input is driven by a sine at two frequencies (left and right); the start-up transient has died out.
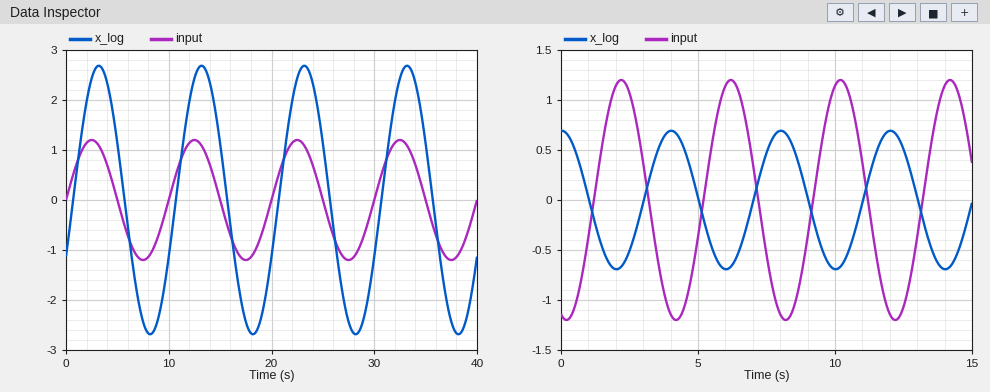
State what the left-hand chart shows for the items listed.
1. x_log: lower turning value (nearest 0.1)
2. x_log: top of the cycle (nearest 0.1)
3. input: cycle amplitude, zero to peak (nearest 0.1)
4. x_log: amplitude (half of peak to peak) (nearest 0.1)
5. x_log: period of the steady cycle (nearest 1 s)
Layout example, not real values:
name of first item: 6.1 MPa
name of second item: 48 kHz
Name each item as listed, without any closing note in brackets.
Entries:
x_log: lower turning value: -2.7
x_log: top of the cycle: 2.7
input: cycle amplitude, zero to peak: 1.2
x_log: amplitude (half of peak to peak): 2.7
x_log: period of the steady cycle: 10 s
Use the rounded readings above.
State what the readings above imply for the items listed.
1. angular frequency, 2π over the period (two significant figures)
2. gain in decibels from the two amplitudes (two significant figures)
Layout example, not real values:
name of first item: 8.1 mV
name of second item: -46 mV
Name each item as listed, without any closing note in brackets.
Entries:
angular frequency, 2π over the period: 0.63 rad/s
gain in decibels from the two amplitudes: 7.0 dB
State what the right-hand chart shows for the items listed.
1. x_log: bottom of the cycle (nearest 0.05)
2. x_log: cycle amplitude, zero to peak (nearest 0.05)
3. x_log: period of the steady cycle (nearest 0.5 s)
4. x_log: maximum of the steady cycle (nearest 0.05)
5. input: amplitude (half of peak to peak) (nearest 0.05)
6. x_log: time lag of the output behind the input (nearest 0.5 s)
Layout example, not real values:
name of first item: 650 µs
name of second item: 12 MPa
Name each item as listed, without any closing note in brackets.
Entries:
x_log: bottom of the cycle: -0.70
x_log: cycle amplitude, zero to peak: 0.70
x_log: period of the steady cycle: 4.0 s
x_log: maximum of the steady cycle: 0.70
input: amplitude (half of peak to peak): 1.20
x_log: time lag of the output behind the input: 2.0 s
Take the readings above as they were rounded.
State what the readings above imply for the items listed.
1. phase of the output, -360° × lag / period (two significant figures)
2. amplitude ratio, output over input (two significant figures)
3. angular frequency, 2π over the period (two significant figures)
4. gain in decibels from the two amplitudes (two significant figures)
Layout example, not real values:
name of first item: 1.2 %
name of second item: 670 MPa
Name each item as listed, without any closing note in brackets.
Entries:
phase of the output, -360° × lag / period: -180°
amplitude ratio, output over input: 0.58
angular frequency, 2π over the period: 1.6 rad/s
gain in decibels from the two amplitudes: -4.7 dB
